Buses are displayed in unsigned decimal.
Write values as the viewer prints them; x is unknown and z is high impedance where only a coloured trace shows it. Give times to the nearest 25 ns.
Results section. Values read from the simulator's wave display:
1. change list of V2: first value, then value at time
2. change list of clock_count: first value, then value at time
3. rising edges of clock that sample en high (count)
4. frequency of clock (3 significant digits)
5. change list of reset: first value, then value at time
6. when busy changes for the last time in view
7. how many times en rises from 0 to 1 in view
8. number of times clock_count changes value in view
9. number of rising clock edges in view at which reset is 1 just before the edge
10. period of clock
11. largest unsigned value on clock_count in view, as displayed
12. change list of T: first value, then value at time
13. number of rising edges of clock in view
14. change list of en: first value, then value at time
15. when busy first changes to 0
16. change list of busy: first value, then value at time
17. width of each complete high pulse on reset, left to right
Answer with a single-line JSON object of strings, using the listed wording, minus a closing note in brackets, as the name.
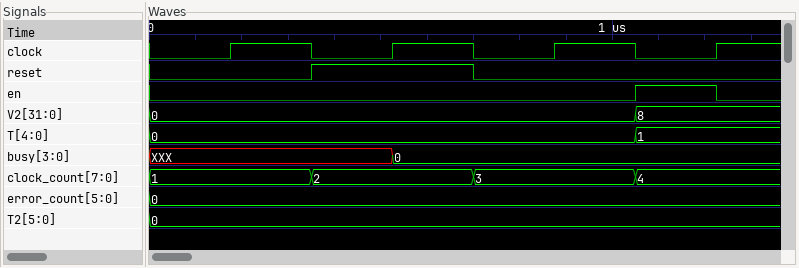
{"change list of V2: first value, then value at time": "0, 8 at 1050 ns", "change list of clock_count: first value, then value at time": "1, 2 at 350 ns, 3 at 700 ns, 4 at 1050 ns", "rising edges of clock that sample en high": "1", "frequency of clock": "2.86 MHz", "change list of reset: first value, then value at time": "0, 1 at 350 ns, 0 at 700 ns", "when busy changes for the last time in view": "525 ns", "how many times en rises from 0 to 1 in view": "1", "number of times clock_count changes value in view": "3", "number of rising clock edges in view at which reset is 1 just before the edge": "1", "period of clock": "350 ns", "largest unsigned value on clock_count in view, as displayed": "4", "change list of T: first value, then value at time": "0, 1 at 1050 ns", "number of rising edges of clock in view": "4", "change list of en: first value, then value at time": "0, 1 at 1050 ns, 0 at 1225 ns", "when busy first changes to 0": "525 ns", "change list of busy: first value, then value at time": "XXX, 0 at 525 ns", "width of each complete high pulse on reset, left to right": "350 ns"}
